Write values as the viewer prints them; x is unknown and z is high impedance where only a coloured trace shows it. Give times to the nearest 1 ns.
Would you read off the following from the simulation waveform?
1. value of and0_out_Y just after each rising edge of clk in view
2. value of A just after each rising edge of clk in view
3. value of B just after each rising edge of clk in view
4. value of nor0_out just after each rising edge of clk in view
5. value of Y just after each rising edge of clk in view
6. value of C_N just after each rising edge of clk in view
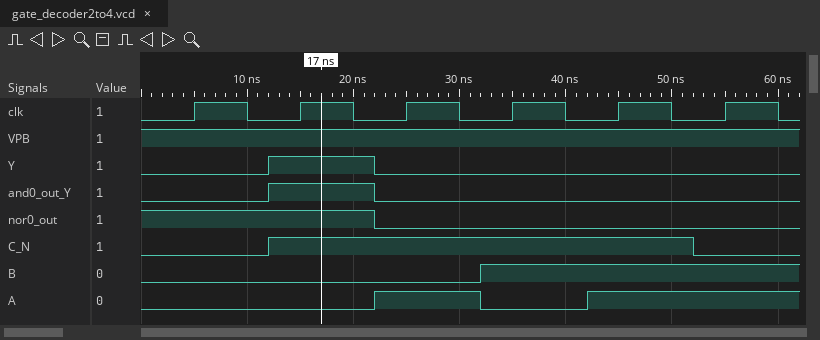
0 1 0 0 0 0
0 0 1 0 1 1
0 0 0 1 1 1
1 1 0 0 0 0
0 1 0 0 0 0
0 1 1 1 1 0
